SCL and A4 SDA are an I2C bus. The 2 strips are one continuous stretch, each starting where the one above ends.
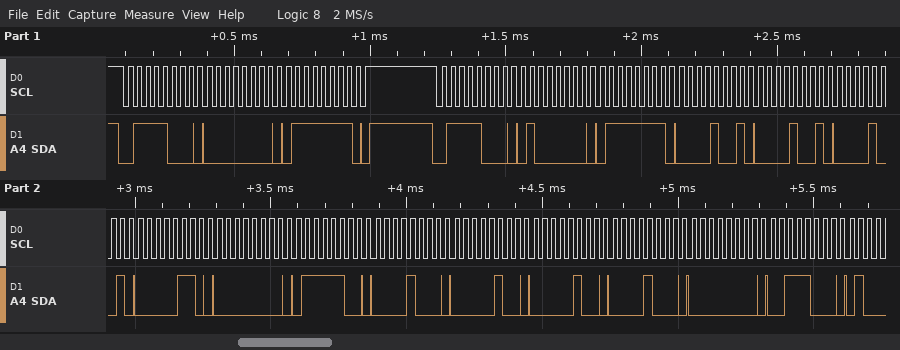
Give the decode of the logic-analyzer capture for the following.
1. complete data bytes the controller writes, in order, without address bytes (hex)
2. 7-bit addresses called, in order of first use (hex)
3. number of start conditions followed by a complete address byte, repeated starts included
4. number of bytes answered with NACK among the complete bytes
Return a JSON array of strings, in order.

["00 7F 40 7F 09 09 09 06 00 7C 08 04 04 08 00 38", "0x3C", "2", "0"]
